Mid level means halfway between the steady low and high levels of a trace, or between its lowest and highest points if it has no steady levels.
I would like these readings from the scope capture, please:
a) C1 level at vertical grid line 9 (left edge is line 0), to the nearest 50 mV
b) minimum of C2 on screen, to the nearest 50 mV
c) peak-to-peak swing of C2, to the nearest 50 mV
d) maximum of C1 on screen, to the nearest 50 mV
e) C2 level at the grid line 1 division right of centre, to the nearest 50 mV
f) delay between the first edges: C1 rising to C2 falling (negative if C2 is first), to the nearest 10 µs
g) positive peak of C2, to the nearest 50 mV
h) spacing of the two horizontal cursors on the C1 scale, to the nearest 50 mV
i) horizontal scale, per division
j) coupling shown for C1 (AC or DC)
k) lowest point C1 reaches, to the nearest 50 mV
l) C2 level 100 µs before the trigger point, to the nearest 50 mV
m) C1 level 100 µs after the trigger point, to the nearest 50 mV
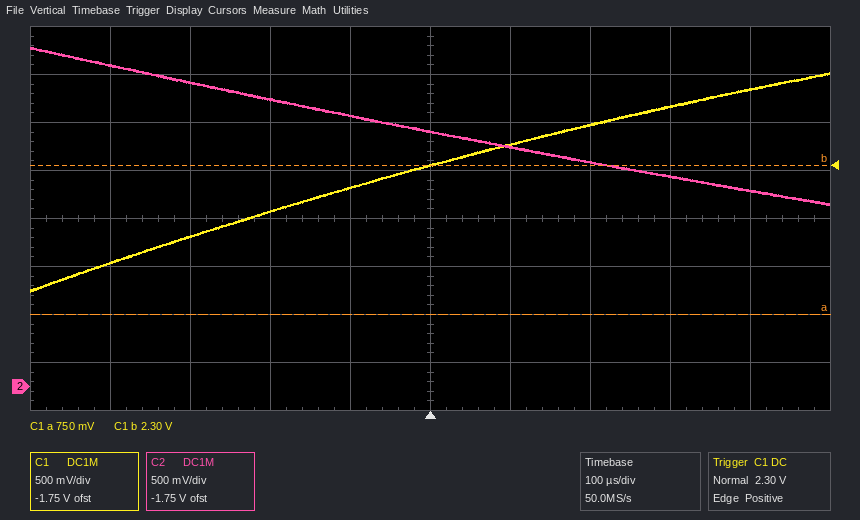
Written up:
3.10 V
1.90 V
1.65 V
3.25 V
2.50 V
+40 µs
3.55 V
1.55 V
100 µs
DC
1.00 V
2.80 V
2.50 V
